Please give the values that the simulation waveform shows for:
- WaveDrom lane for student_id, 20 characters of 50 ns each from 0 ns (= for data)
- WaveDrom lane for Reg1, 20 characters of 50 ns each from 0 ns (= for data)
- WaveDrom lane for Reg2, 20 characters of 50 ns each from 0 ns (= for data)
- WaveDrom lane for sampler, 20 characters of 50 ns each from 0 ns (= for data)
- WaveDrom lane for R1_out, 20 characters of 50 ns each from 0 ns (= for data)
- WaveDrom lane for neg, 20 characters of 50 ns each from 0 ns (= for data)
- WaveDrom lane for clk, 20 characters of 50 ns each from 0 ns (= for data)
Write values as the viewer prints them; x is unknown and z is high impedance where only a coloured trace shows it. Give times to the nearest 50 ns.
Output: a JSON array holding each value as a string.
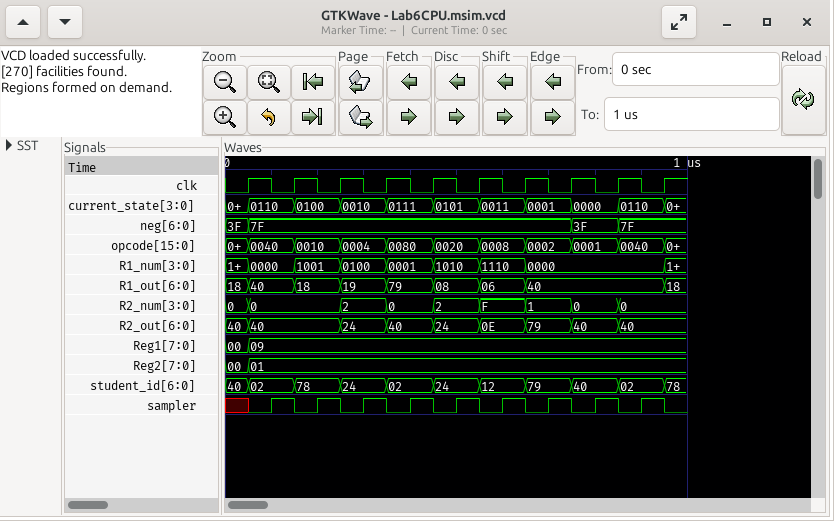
["{name: 'student_id', wave: '==.=.=.=.=.=.=.=.=.=', data: '40 02 78 24 02 24 12 79 40 02 78'}", "{name: 'Reg1', wave: '==..................', data: '00 09'}", "{name: 'Reg2', wave: '==..................', data: '00 01'}", "{name: 'sampler', wave: 'x0101010101010101010'}", "{name: 'R1_out', wave: '==.=.=.=.=.=.=.....=', data: '18 40 18 19 79 08 06 40 18'}", "{name: 'neg', wave: '==.............=.=..', data: '3F 7F 3F 7F'}", "{name: 'clk', wave: '01010101010101010101'}"]
